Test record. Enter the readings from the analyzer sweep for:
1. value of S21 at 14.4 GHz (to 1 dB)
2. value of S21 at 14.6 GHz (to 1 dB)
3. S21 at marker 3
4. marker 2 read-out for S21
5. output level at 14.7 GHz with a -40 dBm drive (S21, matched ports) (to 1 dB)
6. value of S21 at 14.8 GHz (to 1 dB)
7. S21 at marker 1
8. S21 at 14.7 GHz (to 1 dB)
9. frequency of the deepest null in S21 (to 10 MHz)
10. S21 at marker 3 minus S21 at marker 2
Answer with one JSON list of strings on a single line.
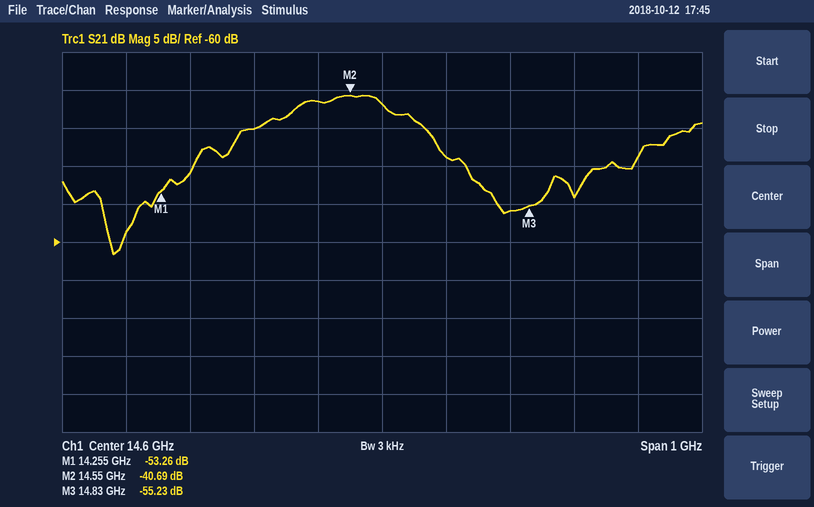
["-45 dB", "-42 dB", "-55.23 dB", "-40.69 dB", "-89 dBm", "-56 dB", "-53.26 dB", "-49 dB", "14.18 GHz", "-14.54 dB"]
